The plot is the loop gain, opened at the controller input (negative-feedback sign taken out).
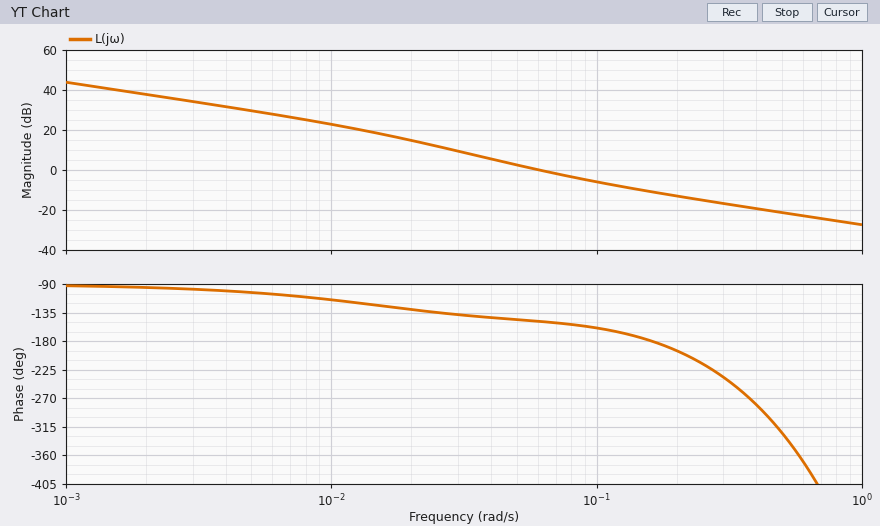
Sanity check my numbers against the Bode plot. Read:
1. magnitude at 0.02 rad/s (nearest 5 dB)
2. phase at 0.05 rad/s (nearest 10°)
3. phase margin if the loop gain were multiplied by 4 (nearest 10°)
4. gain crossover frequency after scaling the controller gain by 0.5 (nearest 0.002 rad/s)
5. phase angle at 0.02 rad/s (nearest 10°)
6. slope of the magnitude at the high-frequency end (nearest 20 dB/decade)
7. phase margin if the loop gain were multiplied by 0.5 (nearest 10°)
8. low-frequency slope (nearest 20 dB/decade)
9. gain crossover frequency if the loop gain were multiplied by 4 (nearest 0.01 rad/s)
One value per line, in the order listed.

15 dB
-150°
-10°
0.038 rad/s
-130°
-20 dB/decade
40°
-20 dB/decade
0.18 rad/s
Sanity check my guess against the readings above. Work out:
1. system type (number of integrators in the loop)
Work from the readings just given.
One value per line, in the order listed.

1
